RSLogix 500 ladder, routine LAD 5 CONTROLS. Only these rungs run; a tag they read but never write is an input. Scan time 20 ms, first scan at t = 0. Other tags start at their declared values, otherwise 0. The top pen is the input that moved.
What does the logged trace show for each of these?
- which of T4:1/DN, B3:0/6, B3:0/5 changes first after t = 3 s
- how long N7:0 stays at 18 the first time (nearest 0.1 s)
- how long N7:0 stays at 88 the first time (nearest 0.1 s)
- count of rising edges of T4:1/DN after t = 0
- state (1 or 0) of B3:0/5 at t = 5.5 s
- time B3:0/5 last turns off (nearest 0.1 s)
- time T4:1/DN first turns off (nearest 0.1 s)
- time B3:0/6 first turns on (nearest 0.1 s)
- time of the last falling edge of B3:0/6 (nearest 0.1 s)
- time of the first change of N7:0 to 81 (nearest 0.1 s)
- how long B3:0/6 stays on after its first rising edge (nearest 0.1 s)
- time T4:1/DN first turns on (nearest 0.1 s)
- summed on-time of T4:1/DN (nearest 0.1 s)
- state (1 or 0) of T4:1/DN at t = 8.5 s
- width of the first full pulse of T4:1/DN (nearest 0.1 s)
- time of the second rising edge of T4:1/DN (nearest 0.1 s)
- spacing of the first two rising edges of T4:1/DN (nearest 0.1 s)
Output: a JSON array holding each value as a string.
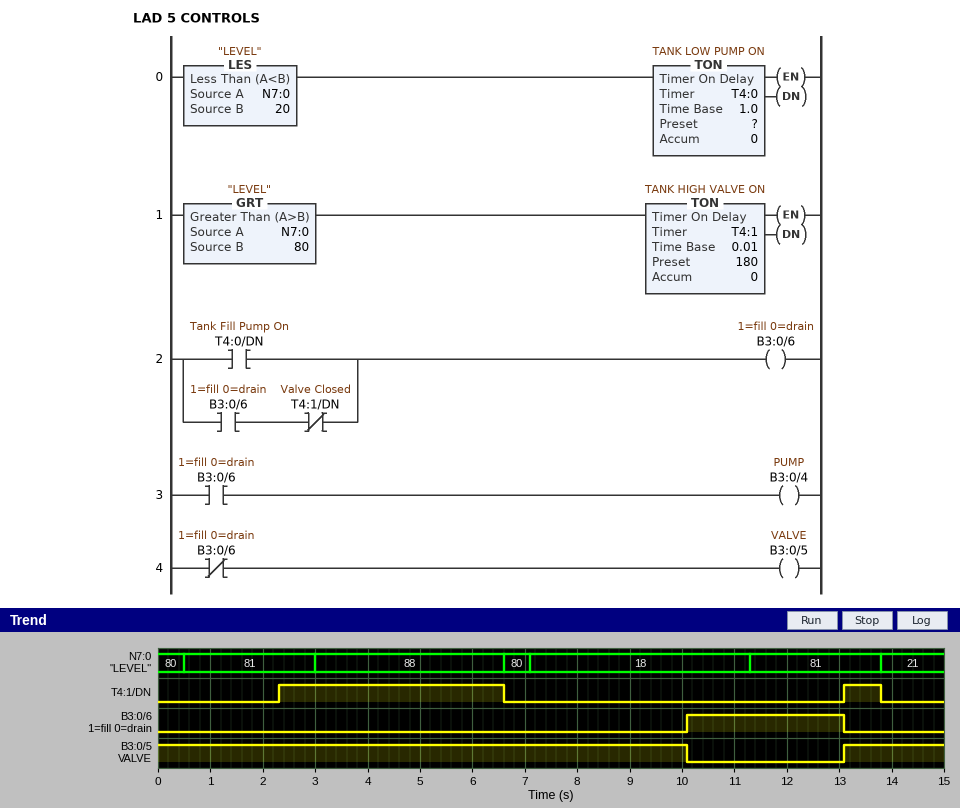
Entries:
["T4:1/DN", "4.2 s", "3.6 s", "2", "1", "10.1 s", "6.6 s", "10.1 s", "13.1 s", "0.5 s", "3.0 s", "2.3 s", "5.0 s", "0", "4.3 s", "13.1 s", "10.8 s"]
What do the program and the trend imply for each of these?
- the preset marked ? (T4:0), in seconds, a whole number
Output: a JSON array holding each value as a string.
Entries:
["3 s"]
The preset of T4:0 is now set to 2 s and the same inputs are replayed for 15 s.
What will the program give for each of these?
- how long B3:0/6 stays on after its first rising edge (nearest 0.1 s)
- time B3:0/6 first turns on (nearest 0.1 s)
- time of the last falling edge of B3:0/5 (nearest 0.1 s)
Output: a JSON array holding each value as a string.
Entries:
["4.0 s", "9.1 s", "9.1 s"]
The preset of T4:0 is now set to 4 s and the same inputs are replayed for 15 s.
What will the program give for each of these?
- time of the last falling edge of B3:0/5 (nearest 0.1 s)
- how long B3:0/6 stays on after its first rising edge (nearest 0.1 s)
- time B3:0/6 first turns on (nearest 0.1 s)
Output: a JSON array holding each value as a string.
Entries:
["11.1 s", "2.0 s", "11.1 s"]
